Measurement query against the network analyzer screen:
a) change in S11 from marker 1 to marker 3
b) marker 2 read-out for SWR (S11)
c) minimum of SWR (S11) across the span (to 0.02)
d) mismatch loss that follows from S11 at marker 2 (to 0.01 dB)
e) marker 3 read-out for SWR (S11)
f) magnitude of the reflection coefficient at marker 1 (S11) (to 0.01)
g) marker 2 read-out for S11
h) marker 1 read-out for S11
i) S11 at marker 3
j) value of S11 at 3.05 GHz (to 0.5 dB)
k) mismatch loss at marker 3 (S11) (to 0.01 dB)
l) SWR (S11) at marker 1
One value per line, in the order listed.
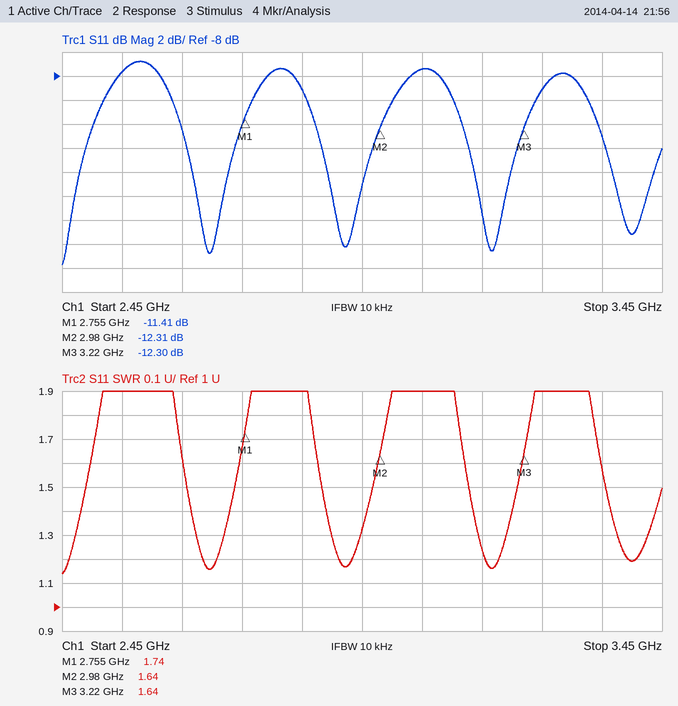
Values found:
-0.89 dB
1.64
1.14
0.26 dB
1.64
0.27
-12.31 dB
-11.41 dB
-12.30 dB
-7.5 dB
0.26 dB
1.74
